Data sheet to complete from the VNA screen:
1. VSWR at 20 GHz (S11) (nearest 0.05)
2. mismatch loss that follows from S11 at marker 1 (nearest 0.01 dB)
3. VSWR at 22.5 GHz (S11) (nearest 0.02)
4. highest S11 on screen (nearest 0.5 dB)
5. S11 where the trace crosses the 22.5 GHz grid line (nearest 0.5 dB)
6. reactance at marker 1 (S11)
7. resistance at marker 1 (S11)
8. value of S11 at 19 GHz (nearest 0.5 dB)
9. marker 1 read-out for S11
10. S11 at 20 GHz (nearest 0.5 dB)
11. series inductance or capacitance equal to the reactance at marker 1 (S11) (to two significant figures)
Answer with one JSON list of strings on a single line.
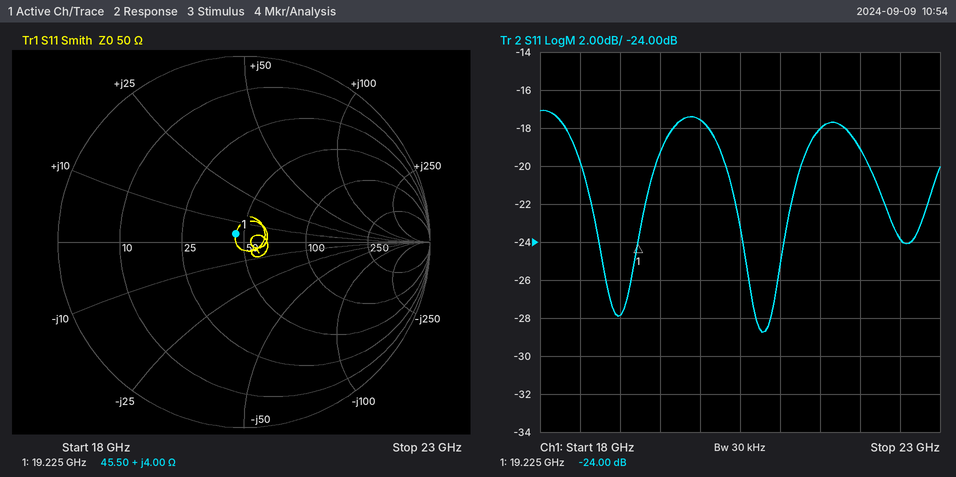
["1.30", "0.02 dB", "1.14", "-17.0 dB", "-24.0 dB", "+4.00 Ω", "45.50 Ω", "-28.0 dB", "-24.00 dB", "-17.5 dB", "33 pH"]
